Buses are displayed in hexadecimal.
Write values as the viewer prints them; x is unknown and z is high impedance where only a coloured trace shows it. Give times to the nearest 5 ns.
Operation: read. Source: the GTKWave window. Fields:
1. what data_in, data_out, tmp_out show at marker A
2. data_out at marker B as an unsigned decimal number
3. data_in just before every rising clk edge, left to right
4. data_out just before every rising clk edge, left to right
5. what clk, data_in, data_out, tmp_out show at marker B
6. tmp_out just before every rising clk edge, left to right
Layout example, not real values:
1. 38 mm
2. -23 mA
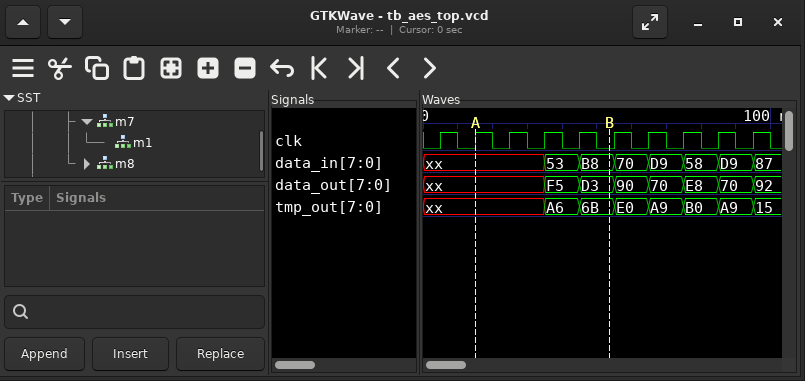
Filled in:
1. data_in=xx, data_out=xx, tmp_out=xx
2. 211
3. xx, xx, xx, xx, 53, B8, 70, D9, 58, D9
4. xx, xx, xx, xx, F5, D3, 90, 70, E8, 70
5. clk=0, data_in=B8, data_out=D3, tmp_out=6B
6. xx, xx, xx, xx, A6, 6B, E0, A9, B0, A9
